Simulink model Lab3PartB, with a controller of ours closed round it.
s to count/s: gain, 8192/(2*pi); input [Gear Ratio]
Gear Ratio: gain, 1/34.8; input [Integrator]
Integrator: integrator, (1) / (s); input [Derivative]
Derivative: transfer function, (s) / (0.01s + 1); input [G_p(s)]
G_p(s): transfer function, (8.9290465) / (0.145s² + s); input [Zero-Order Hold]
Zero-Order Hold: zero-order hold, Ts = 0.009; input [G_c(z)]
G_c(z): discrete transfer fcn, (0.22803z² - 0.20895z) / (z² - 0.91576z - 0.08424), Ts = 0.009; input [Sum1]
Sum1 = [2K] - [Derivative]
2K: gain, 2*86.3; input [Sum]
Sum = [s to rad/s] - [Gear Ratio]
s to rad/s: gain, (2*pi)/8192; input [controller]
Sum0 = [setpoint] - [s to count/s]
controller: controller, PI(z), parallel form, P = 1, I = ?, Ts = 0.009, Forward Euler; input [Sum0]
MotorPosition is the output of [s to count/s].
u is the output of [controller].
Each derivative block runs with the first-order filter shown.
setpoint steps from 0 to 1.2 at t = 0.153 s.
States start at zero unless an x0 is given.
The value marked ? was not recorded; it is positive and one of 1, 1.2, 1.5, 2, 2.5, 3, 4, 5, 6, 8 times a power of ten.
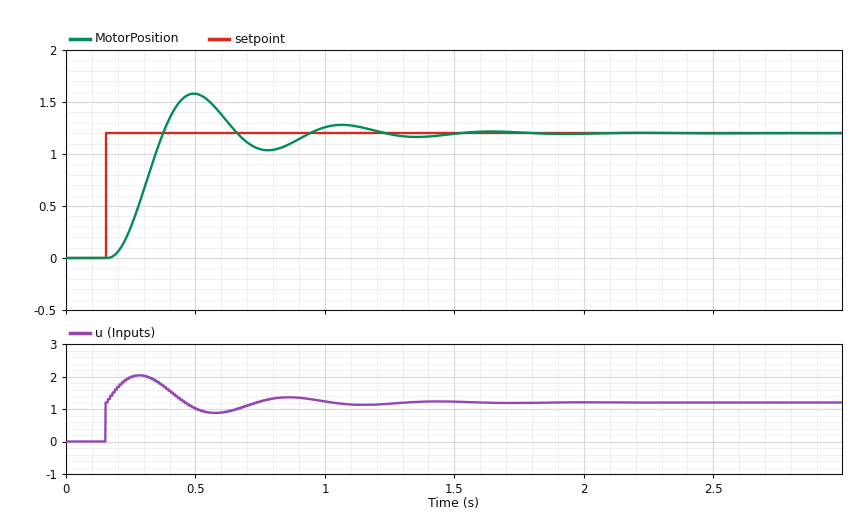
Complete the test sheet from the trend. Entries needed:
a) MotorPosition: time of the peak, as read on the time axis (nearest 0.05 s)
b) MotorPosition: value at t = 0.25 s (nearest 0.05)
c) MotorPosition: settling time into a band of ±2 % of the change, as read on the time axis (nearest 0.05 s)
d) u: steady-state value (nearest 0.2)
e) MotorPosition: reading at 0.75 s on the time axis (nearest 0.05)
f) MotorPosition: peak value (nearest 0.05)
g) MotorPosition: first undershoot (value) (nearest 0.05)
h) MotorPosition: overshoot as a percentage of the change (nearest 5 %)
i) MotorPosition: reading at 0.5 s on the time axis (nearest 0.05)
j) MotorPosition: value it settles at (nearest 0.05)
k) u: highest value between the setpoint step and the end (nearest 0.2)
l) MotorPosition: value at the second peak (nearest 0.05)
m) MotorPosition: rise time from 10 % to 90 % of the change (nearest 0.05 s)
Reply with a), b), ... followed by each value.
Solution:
a) 0.50 s
b) 0.30
c) 1.45 s
d) 1.2
e) 1.05
f) 1.60
g) 1.05
h) 30 %
i) 1.60
j) 1.20
k) 2.0
l) 1.30
m) 0.15 s
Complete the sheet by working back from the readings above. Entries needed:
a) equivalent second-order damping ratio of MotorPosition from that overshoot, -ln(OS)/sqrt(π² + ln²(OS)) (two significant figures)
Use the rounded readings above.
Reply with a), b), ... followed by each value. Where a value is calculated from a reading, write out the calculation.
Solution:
a) ln(0.3) = -1.204; 1.204 / sqrt(9.870 + 1.450) = 0.36
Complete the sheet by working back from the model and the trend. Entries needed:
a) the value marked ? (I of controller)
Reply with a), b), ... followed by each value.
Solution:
a) 10
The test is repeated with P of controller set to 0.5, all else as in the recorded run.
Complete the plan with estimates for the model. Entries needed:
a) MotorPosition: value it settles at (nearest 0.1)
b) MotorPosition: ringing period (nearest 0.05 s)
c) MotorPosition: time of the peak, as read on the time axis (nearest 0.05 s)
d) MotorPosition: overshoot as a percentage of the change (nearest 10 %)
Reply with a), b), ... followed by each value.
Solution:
a) 1.2
b) 0.70 s
c) 0.55 s
d) 50 %
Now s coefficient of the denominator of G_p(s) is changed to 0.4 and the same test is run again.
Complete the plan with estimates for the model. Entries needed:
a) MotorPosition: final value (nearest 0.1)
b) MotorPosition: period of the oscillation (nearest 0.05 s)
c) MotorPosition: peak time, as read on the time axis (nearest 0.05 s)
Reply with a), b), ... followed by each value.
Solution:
a) 1.2
b) 0.45 s
c) 0.45 s
